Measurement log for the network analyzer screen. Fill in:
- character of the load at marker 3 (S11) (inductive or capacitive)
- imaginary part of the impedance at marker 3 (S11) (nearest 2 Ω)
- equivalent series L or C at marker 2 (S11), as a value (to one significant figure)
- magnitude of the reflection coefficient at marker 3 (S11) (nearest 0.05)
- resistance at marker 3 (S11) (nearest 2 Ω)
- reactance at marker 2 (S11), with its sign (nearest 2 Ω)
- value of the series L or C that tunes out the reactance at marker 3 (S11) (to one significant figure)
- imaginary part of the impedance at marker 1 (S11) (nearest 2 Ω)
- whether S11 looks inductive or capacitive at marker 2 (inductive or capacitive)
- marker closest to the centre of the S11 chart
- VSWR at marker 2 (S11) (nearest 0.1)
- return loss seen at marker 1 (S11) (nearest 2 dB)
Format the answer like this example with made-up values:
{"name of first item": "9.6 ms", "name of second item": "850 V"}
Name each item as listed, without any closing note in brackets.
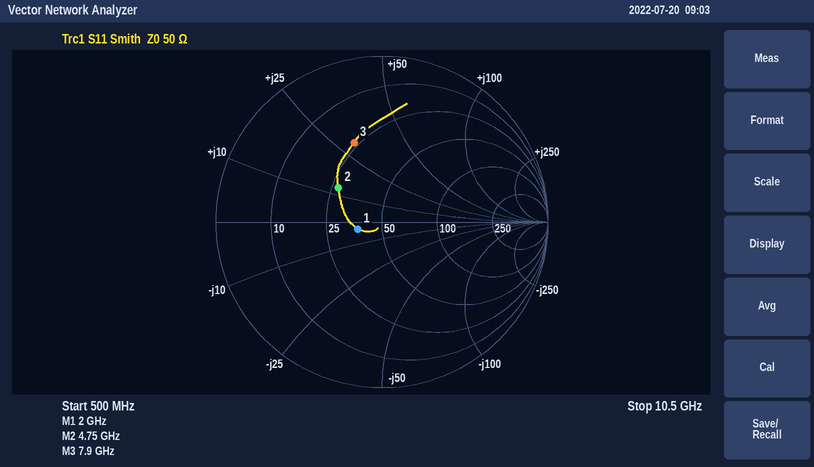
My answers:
{"character of the load at marker 3 (S11)": "inductive", "imaginary part of the impedance at marker 3 (S11)": "+30 Ω", "equivalent series L or C at marker 2 (S11), as a value": "400 pH", "magnitude of the reflection coefficient at marker 3 (S11)": "0.50", "resistance at marker 3 (S11)": "24 Ω", "reactance at marker 2 (S11), with its sign": "+12 Ω", "value of the series L or C that tunes out the reactance at marker 3 (S11)": "700 fF", "imaginary part of the impedance at marker 1 (S11)": "-4 Ω", "whether S11 looks inductive or capacitive at marker 2": "inductive", "marker closest to the centre of the S11 chart": "marker 1", "VSWR at marker 2 (S11)": "2.0", "return loss seen at marker 1 (S11)": "16 dB"}
